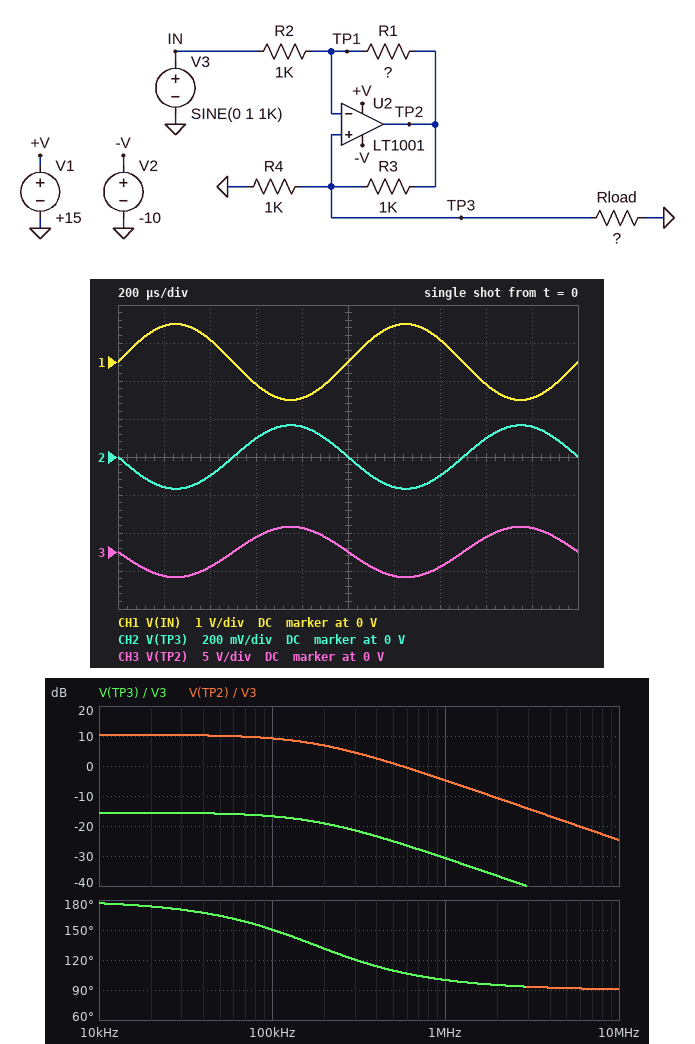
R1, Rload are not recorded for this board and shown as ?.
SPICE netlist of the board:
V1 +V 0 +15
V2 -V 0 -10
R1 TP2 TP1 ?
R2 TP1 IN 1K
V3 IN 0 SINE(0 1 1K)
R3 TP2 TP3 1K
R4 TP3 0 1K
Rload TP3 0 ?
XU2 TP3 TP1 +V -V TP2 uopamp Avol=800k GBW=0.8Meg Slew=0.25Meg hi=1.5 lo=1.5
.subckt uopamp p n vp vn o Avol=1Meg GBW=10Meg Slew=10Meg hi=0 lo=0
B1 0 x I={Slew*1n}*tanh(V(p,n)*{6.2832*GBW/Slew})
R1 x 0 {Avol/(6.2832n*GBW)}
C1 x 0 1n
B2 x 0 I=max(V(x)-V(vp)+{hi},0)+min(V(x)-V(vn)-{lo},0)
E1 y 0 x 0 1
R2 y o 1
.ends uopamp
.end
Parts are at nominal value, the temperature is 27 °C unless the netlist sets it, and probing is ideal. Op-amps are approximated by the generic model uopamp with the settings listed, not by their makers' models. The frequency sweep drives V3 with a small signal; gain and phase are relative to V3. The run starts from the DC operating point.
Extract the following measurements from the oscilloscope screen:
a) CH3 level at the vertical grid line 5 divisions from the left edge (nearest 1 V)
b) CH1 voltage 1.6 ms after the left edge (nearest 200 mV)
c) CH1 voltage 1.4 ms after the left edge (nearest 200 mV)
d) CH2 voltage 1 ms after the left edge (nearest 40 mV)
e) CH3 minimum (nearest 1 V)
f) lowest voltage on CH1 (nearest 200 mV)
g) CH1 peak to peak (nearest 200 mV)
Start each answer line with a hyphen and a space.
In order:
- 0 V
- -600 mV
- 600 mV
- 0 V
- -3 V
- -1.0 V
- 2.0 V
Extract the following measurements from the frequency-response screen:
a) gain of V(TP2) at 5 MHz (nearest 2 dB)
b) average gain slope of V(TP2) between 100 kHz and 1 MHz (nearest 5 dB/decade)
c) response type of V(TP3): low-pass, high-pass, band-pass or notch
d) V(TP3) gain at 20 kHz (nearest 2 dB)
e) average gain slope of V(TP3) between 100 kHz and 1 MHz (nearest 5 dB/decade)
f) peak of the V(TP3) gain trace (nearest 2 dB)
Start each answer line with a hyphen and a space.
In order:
- -18 dB
- -15 dB/decade
- low-pass
- -16 dB
- -15 dB/decade
- -16 dB
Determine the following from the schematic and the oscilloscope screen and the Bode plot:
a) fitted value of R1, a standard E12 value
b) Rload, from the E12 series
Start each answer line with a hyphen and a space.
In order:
- 2.7 kΩ
- 56 Ω
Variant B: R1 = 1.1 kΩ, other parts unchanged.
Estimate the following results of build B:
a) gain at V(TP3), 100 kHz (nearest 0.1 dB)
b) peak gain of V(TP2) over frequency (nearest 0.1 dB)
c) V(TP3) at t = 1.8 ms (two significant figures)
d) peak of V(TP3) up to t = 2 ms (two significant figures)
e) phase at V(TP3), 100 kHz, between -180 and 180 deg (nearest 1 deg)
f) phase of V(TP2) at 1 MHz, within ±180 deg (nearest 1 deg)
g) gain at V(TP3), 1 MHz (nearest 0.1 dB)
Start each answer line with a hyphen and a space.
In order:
- -24.5 dB
- 1.8 dB
- 59 mV
- 62 mV
- 164 deg
- 109 deg
- -34.0 dB
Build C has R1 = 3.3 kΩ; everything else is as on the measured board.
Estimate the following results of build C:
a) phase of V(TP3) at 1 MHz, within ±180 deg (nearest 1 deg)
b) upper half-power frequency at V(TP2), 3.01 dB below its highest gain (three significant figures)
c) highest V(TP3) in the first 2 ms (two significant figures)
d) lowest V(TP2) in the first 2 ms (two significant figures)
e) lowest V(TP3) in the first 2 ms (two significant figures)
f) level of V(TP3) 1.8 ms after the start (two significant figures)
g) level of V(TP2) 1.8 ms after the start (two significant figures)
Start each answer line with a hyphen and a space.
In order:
- 98 deg
- 146 kHz
- 210 mV
- -4.2 V
- -210 mV
- 200 mV
- 4.0 V
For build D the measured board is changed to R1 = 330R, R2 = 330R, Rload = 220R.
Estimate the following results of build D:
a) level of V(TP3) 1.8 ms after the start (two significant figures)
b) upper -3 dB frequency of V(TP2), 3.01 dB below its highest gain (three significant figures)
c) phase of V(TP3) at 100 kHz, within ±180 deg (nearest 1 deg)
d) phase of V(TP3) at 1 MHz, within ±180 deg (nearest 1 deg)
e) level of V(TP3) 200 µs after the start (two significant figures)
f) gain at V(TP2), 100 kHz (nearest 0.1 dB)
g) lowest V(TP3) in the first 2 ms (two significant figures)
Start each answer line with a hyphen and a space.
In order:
- 210 mV
- 277 kHz
- 160 deg
- 105 deg
- -210 mV
- 2.6 dB
- -220 mV
